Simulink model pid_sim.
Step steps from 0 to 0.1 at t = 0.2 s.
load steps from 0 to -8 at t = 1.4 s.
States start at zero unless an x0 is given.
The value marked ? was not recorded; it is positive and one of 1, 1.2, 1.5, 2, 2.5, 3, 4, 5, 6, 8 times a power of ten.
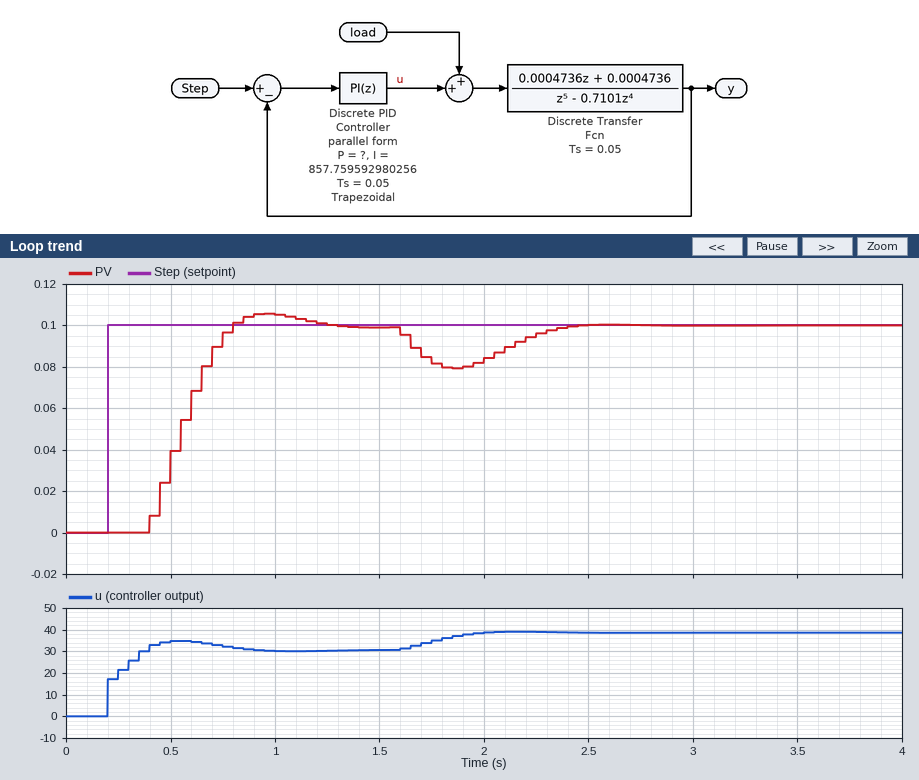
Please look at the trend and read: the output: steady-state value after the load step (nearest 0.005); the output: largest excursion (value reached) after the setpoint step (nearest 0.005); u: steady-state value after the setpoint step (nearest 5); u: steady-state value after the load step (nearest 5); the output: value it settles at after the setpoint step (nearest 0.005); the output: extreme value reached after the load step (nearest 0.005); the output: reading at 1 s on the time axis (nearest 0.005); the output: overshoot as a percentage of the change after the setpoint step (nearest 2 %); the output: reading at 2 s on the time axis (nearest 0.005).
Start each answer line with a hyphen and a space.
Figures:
- 0.100
- 0.105
- 30
- 40
- 0.100
- 0.080
- 0.105
- 6 %
- 0.085
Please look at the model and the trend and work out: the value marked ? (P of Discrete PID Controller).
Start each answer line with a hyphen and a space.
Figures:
- 150
